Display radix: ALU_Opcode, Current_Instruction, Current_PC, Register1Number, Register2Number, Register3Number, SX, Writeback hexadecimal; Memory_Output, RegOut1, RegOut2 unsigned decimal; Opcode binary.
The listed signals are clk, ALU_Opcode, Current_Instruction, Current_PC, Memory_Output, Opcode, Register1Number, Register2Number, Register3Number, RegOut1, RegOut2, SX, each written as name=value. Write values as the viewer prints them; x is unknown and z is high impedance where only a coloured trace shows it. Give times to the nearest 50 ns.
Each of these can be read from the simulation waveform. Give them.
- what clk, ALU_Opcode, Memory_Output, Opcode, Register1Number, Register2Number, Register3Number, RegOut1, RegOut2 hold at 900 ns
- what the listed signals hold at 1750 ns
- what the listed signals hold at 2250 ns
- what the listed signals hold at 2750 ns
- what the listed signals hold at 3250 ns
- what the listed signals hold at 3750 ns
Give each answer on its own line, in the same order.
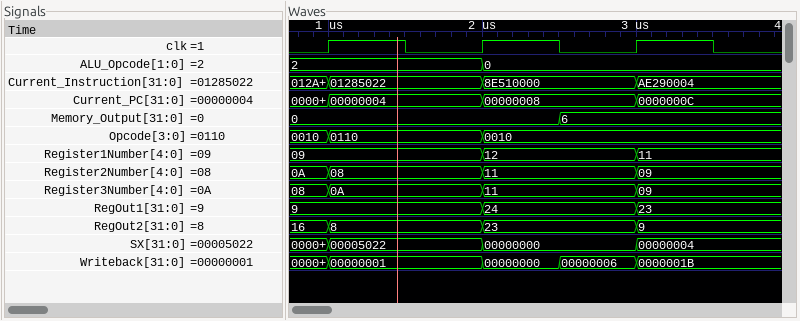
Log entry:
clk=0, ALU_Opcode=2, Memory_Output=0, Opcode=0010, Register1Number=09, Register2Number=0A, Register3Number=08, RegOut1=9, RegOut2=16
clk=0, ALU_Opcode=2, Current_Instruction=01285022, Current_PC=00000004, Memory_Output=0, Opcode=0110, Register1Number=09, Register2Number=08, Register3Number=0A, RegOut1=9, RegOut2=8, SX=00005022
clk=1, ALU_Opcode=0, Current_Instruction=8E510000, Current_PC=00000008, Memory_Output=0, Opcode=0010, Register1Number=12, Register2Number=11, Register3Number=11, RegOut1=24, RegOut2=23, SX=00000000
clk=0, ALU_Opcode=0, Current_Instruction=8E510000, Current_PC=00000008, Memory_Output=6, Opcode=0010, Register1Number=12, Register2Number=11, Register3Number=11, RegOut1=24, RegOut2=23, SX=00000000
clk=1, ALU_Opcode=0, Current_Instruction=AE290004, Current_PC=0000000C, Memory_Output=6, Opcode=0010, Register1Number=11, Register2Number=09, Register3Number=09, RegOut1=23, RegOut2=9, SX=00000004
clk=0, ALU_Opcode=0, Current_Instruction=AE290004, Current_PC=0000000C, Memory_Output=6, Opcode=0010, Register1Number=11, Register2Number=09, Register3Number=09, RegOut1=23, RegOut2=9, SX=00000004
